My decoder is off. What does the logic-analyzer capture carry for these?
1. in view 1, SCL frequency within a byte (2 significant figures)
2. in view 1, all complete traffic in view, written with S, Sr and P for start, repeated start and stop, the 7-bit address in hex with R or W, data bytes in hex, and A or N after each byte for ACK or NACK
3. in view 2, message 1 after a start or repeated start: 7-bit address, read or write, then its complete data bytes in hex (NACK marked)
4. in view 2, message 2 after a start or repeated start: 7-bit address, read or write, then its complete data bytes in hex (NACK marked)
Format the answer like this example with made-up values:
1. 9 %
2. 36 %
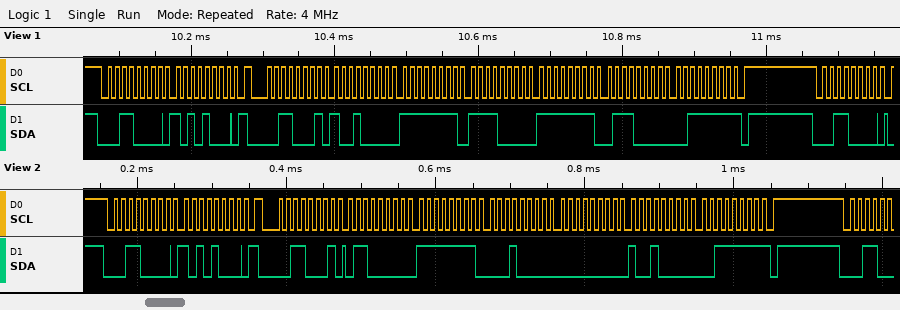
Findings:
1. 100 kHz
2. S 18W A A8 A Sr 18R A 90 A FF A F0 A FF A 70 A 3F N P S 18W A
3. 0x18 write: A8
4. 0x18 read: 60 FF 10 00 90 3F NACK
